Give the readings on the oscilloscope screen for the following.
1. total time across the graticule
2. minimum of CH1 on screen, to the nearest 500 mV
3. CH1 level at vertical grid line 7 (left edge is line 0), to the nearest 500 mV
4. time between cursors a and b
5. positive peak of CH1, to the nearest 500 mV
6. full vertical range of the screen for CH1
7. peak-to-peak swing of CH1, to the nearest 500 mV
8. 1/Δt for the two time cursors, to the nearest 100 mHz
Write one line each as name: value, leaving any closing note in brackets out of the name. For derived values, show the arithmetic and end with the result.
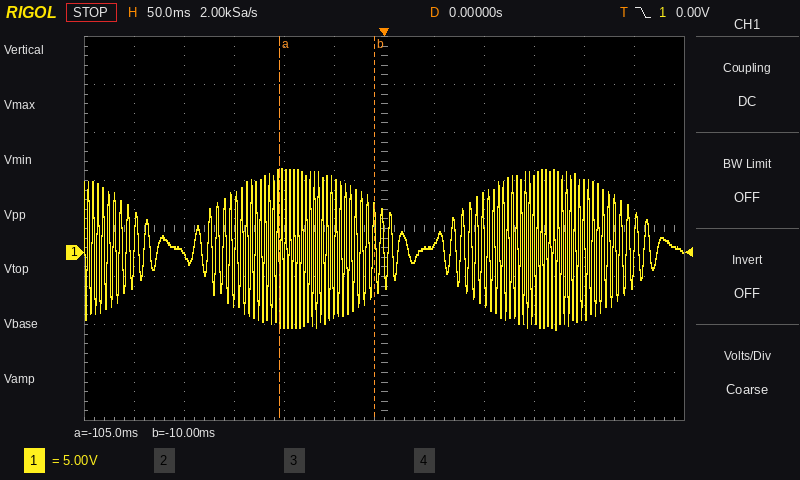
total time across the graticule: 600 ms
minimum of CH1 on screen, to the nearest 500 mV: -8.0 V
CH1 level at vertical grid line 7 (left edge is line 0), to the nearest 500 mV: 1.0 V
time between cursors a and b: -10 ms − (-105 ms) = 95 ms
positive peak of CH1, to the nearest 500 mV: 9.0 V
full vertical range of the screen for CH1: 40 V
peak-to-peak swing of CH1, to the nearest 500 mV: 9.0 V − (-8.0 V) = 17.0 V
1/Δt for the two time cursors, to the nearest 100 mHz: 1 / 95 ms ≈ 10.5 Hz
